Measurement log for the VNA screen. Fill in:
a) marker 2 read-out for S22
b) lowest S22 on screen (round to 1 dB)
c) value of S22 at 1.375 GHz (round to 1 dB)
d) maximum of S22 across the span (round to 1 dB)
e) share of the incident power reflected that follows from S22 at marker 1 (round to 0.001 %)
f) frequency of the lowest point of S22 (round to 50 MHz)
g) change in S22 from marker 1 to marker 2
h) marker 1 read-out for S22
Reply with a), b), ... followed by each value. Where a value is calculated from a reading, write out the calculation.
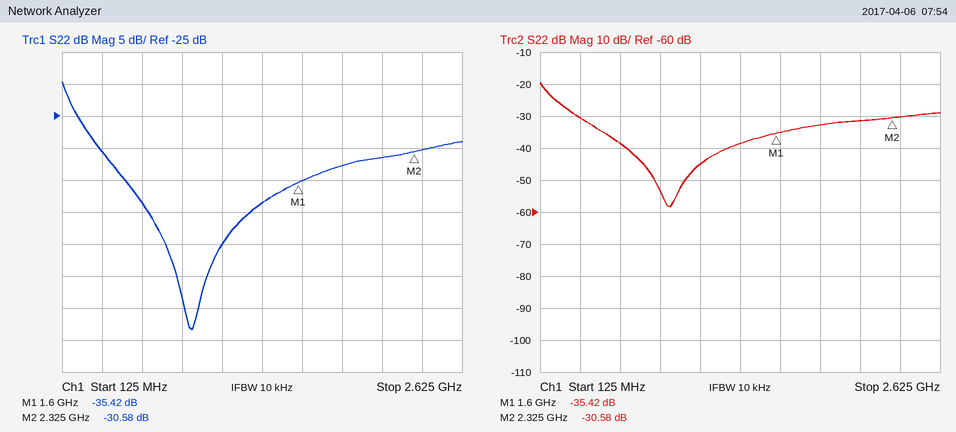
a) -30.58 dB
b) -58 dB
c) -39 dB
d) -20 dB
e) 10^(-35.42/10) ≈ 0.029 %
f) 950 MHz
g) -30.58 − (-35.42) = 4.84 dB
h) -35.42 dB
